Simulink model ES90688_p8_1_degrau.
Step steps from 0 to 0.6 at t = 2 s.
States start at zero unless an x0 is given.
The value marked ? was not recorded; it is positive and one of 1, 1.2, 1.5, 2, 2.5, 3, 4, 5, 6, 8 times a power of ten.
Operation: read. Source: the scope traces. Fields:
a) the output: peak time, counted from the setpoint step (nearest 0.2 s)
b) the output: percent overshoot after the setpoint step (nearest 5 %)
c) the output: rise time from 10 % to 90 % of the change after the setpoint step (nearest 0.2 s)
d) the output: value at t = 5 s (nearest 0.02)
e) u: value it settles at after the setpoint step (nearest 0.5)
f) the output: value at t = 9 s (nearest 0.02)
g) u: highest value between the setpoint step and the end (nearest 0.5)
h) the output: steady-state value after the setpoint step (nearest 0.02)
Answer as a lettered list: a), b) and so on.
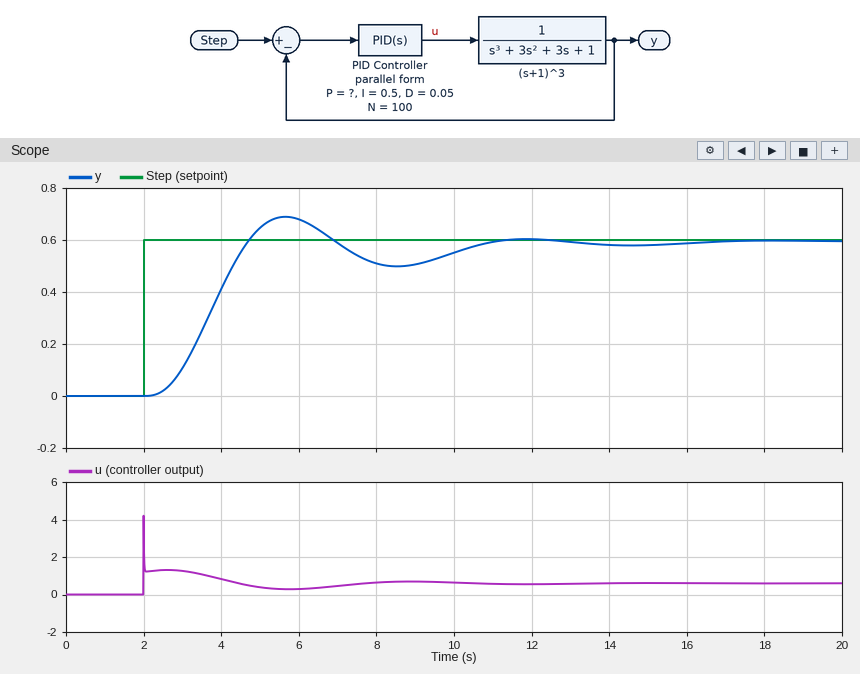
a) 3.6 s
b) 15 %
c) 1.6 s
d) 0.64
e) 0.5
f) 0.50
g) 4.0
h) 0.60
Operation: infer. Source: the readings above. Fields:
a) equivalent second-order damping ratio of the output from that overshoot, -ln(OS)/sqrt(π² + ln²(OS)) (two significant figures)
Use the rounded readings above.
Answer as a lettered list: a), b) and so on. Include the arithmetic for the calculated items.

a) ln(0.15) = -1.897; 1.897 / sqrt(9.870 + 3.599) = 0.52
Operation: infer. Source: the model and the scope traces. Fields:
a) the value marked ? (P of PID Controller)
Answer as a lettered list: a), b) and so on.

a) 2
